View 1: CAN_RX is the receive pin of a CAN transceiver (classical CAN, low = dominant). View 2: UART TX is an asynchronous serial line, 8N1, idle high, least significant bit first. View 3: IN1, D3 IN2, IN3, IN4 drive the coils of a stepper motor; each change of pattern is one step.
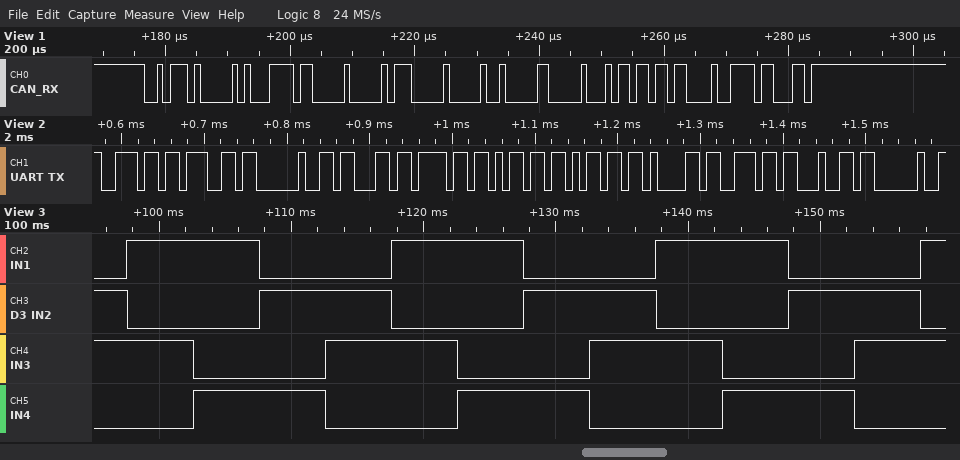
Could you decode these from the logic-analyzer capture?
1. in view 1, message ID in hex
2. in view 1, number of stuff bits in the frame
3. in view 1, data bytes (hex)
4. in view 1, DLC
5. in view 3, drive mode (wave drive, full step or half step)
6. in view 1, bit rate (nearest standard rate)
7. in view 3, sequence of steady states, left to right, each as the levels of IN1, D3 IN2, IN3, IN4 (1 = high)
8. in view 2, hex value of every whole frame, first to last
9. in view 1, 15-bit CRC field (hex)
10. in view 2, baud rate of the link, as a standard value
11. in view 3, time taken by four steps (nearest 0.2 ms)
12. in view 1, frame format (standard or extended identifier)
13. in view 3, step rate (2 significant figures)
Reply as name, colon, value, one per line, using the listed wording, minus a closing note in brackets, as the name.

in view 1, message ID in hex: 0x2E8
in view 1, number of stuff bits in the frame: 7
in view 1, data bytes: F6 00 38 00 41 00 B6 D8
in view 1, DLC: 8
in view 3, drive mode: full step
in view 1, bit rate: 1000 kbit/s
in view 3, sequence of steady states, left to right, each as the levels of IN1, D3 IN2, IN3, IN4: 0110 1010 1001 0101 0110 1010 1001 0101 0110 1010 1001 0101 0110 1010
in view 2, hex value of every whole frame, first to last: 0x6E 0x67 0x20 0x63 0x6F 0x6D 0x6D 0x61 0x6E 0x64 0x20
in view 1, 15-bit CRC field: 0x27B1
in view 2, baud rate of the link, as a standard value: 115200 baud
in view 3, time taken by four steps: 20.0 ms
in view 1, frame format: standard
in view 3, step rate: 200 steps/s
